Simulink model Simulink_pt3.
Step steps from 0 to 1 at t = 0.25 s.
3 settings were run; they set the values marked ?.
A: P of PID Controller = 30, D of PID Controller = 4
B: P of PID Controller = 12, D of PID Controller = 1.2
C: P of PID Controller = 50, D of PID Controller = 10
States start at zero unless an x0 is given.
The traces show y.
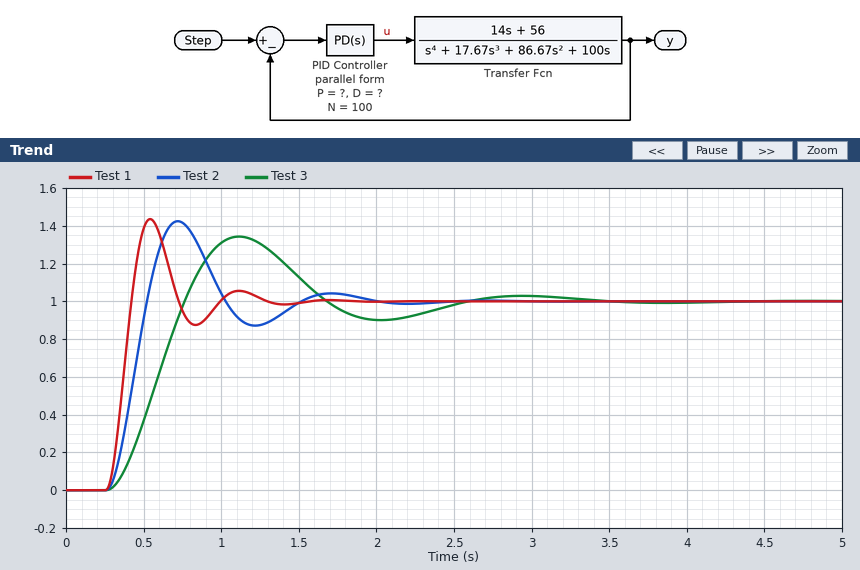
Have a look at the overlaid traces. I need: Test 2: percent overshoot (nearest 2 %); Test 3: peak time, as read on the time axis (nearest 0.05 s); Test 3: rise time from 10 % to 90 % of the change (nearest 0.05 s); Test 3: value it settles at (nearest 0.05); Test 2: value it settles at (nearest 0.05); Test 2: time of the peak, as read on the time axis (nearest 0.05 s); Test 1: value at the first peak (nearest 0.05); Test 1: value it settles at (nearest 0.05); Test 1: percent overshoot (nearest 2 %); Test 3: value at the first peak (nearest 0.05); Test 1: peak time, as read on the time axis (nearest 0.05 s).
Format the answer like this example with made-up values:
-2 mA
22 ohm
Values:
42 %
1.10 s
0.35 s
1.00
1.00
0.70 s
1.45
1.00
44 %
1.35
0.55 s
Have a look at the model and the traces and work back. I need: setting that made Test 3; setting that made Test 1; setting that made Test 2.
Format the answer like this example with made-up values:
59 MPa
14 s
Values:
B
C
A
